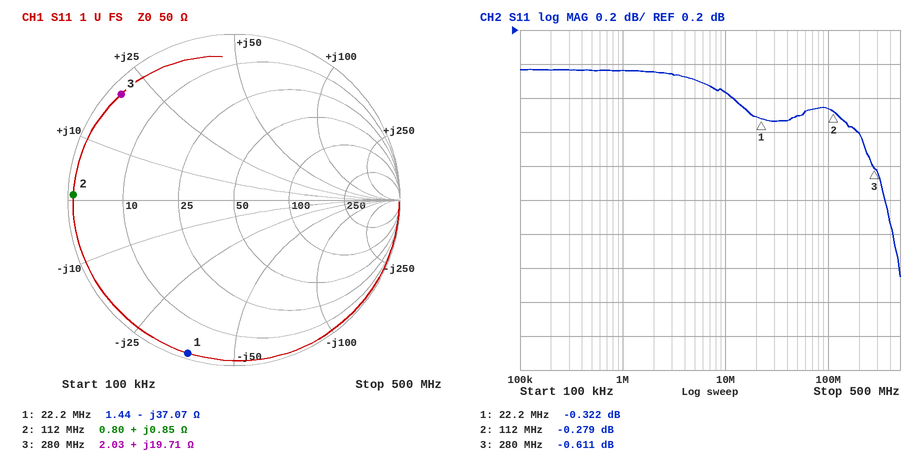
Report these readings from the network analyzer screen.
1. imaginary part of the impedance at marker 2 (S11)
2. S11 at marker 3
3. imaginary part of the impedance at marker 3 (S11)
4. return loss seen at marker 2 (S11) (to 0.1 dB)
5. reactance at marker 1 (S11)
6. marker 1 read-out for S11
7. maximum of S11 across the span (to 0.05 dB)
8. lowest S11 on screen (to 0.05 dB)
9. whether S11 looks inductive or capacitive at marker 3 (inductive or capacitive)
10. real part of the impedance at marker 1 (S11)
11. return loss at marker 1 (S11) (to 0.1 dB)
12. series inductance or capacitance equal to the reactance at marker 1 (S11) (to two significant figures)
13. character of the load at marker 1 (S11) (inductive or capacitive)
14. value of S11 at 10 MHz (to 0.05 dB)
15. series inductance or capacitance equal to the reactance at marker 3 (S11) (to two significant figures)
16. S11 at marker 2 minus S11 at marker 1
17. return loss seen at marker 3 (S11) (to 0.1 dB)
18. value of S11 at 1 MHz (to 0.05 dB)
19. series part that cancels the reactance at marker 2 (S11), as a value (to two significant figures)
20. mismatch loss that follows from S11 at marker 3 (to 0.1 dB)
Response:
+0.85 Ω
-0.611 dB
+19.71 Ω
0.3 dB
-37.07 Ω
-0.322 dB
-0.05 dB
-1.25 dB
inductive
1.44 Ω
0.3 dB
190 pF
capacitive
-0.15 dB
11 nH
0.043 dB
0.6 dB
-0.05 dB
1.7 nF
8.8 dB
